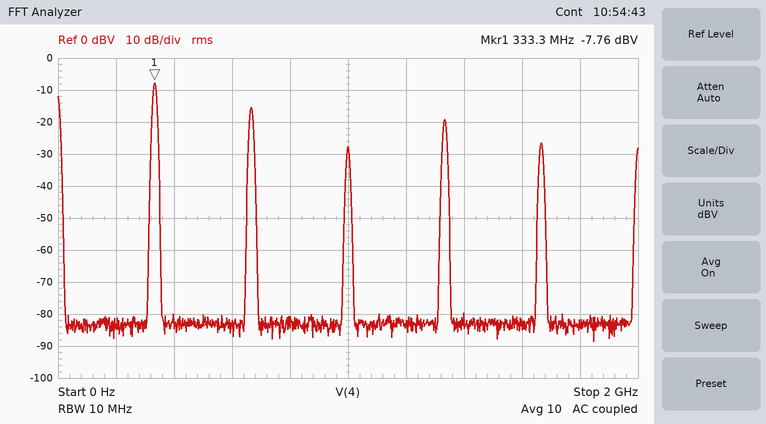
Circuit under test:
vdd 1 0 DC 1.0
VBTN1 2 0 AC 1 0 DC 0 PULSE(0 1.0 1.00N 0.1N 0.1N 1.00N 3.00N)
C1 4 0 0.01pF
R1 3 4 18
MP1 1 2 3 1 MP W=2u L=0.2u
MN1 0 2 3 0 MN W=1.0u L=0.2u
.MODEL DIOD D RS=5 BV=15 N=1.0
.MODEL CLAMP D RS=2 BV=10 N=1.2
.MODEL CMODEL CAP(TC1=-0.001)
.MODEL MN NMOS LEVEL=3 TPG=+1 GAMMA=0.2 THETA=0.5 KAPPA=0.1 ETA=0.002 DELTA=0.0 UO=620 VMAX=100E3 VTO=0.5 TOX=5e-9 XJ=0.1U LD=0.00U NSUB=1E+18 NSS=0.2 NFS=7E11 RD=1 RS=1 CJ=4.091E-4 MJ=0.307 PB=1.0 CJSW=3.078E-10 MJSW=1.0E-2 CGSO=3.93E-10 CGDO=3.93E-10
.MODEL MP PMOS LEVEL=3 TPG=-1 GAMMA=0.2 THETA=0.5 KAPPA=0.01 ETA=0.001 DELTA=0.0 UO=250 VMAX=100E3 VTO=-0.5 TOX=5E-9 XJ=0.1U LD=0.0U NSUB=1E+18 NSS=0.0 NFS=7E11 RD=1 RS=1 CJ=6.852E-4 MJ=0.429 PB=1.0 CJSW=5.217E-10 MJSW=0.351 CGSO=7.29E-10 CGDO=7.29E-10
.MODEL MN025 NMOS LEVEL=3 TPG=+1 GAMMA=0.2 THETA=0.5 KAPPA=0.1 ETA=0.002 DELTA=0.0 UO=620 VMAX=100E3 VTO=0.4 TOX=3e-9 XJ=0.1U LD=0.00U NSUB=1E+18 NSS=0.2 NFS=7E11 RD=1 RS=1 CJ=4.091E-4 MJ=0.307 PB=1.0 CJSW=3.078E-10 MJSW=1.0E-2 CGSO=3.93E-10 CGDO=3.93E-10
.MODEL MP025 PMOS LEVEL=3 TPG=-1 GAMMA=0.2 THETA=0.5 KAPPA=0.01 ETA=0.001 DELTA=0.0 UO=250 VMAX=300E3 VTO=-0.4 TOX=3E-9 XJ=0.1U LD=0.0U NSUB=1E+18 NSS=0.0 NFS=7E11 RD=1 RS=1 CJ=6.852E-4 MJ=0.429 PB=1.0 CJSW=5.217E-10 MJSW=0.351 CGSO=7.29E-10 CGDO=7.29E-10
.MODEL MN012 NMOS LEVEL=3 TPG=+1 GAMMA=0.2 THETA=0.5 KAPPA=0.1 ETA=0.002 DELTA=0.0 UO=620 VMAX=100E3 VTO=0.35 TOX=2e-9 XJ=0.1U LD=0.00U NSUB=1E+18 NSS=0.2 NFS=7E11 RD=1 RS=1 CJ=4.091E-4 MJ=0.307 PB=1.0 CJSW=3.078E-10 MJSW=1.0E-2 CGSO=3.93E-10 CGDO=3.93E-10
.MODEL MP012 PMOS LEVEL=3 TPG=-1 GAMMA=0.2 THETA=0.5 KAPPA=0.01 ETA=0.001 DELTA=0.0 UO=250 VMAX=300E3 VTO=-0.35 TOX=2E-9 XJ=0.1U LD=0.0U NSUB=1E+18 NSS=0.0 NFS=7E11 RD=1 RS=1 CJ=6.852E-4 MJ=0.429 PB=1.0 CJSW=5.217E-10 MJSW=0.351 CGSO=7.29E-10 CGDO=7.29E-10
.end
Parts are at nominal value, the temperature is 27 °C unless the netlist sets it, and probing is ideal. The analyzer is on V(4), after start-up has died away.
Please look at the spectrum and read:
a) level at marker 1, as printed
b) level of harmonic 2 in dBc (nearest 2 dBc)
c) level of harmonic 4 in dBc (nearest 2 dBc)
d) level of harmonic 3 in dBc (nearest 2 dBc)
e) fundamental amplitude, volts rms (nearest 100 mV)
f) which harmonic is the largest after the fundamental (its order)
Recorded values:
-7.76 dBV
-8 dBc
-12 dBc
-20 dBc
400 mV
2
